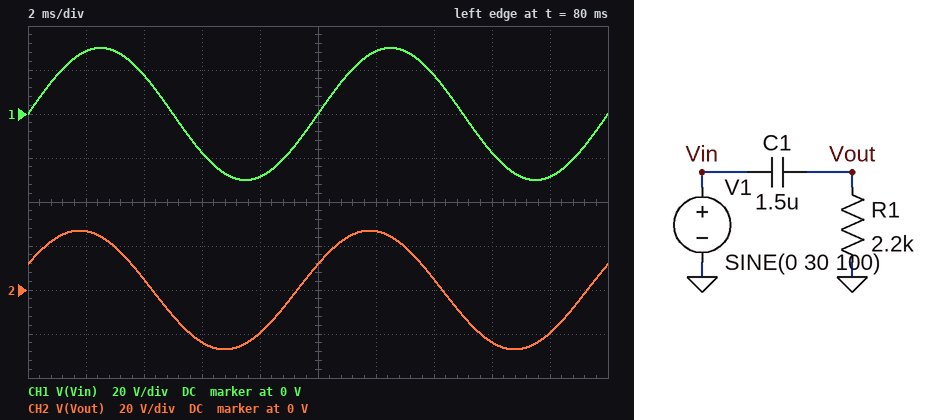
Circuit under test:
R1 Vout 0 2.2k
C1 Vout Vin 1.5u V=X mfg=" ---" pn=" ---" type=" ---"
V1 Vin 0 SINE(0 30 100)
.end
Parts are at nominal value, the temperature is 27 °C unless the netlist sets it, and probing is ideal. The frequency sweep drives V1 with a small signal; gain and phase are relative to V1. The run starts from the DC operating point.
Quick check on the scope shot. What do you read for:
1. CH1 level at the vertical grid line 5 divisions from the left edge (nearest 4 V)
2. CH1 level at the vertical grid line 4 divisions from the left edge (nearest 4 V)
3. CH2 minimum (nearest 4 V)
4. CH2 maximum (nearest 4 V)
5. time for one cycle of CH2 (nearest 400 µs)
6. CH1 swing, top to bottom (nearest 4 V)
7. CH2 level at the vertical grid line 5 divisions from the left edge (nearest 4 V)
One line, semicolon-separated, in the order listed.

0 V; -28 V; -28 V; 28 V; 10.0 ms; 60 V; 12 V
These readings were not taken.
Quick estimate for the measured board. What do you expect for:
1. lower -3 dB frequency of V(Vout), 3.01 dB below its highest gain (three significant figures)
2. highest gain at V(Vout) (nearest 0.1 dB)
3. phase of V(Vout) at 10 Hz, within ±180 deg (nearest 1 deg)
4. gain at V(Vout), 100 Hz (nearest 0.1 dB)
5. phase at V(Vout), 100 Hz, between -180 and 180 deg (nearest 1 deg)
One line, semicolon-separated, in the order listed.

48.2 Hz; 0 dB; 78 deg; -0.9 dB; 26 deg
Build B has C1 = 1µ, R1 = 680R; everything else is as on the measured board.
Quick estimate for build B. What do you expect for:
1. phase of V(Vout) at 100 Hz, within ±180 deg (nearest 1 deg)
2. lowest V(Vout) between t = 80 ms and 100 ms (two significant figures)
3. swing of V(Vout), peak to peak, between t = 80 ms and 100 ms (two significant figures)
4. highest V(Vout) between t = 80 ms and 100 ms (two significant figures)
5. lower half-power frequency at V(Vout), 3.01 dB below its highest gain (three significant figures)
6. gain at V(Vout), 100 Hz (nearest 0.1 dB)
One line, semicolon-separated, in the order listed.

67 deg; -12 V; 24 V; 12 V; 234 Hz; -8.1 dB
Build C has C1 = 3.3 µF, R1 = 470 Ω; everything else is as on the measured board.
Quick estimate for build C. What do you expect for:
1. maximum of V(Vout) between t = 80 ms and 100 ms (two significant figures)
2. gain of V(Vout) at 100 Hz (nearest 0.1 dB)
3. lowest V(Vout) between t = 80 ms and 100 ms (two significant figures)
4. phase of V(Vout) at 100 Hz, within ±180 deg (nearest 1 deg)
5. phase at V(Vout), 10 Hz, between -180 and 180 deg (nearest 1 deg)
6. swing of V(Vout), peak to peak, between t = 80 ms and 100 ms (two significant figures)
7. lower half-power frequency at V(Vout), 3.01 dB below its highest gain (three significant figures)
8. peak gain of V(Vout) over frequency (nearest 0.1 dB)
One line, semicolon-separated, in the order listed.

21 V; -3.1 dB; -21 V; 46 deg; 84 deg; 42 V; 103 Hz; 0 dB
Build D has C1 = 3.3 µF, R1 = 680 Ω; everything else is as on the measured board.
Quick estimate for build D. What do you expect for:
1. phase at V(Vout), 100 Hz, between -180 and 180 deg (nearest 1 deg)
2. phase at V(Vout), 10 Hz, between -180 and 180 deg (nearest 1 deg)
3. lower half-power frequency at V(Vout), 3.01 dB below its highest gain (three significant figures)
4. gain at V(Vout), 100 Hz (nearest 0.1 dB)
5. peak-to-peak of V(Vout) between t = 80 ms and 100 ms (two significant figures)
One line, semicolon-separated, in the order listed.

35 deg; 82 deg; 70.9 Hz; -1.8 dB; 49 V
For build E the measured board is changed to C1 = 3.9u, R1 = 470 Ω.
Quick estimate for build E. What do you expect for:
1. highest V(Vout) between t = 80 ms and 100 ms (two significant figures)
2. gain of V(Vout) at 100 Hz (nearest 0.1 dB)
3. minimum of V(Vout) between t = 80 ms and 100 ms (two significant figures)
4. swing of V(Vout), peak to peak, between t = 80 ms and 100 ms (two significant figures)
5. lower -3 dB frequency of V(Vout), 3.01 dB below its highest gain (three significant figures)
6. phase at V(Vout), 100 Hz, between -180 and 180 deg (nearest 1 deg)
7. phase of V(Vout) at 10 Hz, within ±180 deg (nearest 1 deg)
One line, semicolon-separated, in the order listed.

23 V; -2.4 dB; -23 V; 45 V; 86.8 Hz; 41 deg; 83 deg
